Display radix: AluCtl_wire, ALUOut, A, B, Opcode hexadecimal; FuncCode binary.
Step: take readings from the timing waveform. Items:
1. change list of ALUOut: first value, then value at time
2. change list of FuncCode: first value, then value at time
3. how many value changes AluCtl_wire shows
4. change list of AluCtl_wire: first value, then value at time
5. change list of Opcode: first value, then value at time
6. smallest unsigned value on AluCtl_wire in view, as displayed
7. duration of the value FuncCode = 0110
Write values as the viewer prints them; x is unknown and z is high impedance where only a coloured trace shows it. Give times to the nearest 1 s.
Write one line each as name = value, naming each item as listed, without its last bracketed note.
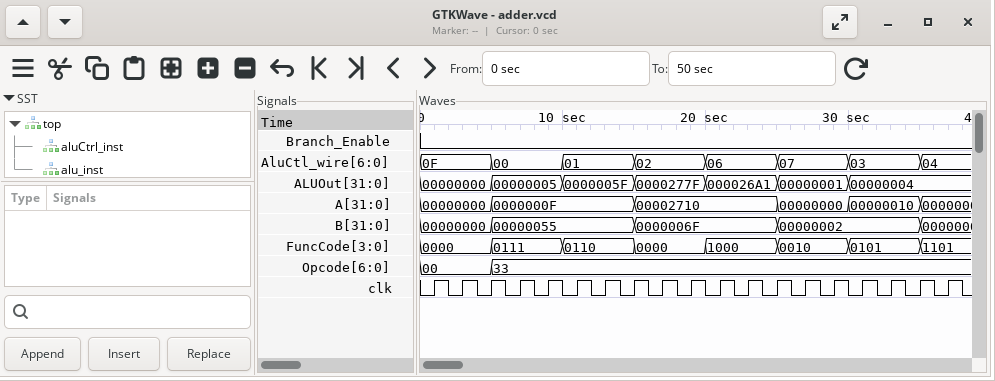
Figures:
change list of ALUOut: first value, then value at time = 00000000, 00000005 at 5 s, 0000005F at 10 s, 0000277F at 15 s, 000026A1 at 20 s, 00000001 at 25 s, 00000004 at 30 s
change list of FuncCode: first value, then value at time = 0000, 0111 at 5 s, 0110 at 10 s, 0000 at 15 s, 1000 at 20 s, 0010 at 25 s, 0101 at 30 s, 1101 at 35 s
how many value changes AluCtl_wire shows = 7
change list of AluCtl_wire: first value, then value at time = 0F, 00 at 5 s, 01 at 10 s, 02 at 15 s, 06 at 20 s, 07 at 25 s, 03 at 30 s, 04 at 35 s
change list of Opcode: first value, then value at time = 00, 33 at 5 s
smallest unsigned value on AluCtl_wire in view, as displayed = 00
duration of the value FuncCode = 0110 = 5 s
